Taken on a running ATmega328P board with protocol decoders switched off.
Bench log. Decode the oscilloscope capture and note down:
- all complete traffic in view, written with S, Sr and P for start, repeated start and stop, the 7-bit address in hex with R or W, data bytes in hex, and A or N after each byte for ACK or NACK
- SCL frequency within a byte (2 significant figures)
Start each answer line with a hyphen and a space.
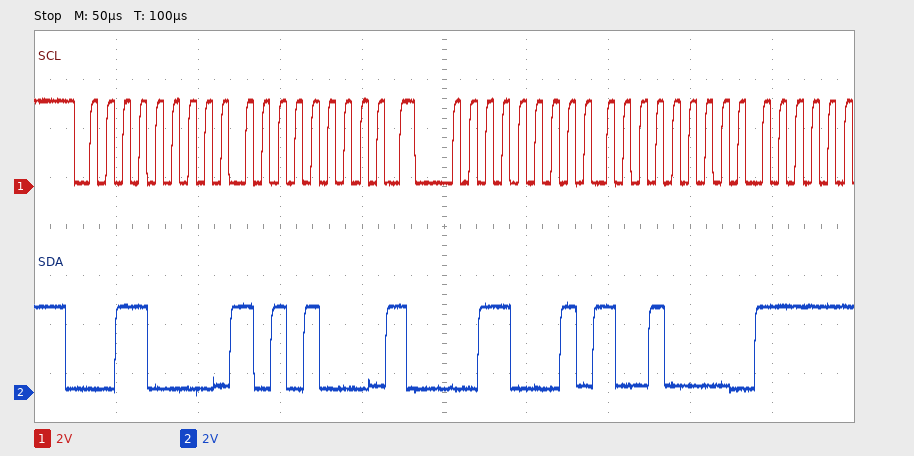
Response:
- S 18W A A8 A Sr 18R A 90 A
- 100 kHz
